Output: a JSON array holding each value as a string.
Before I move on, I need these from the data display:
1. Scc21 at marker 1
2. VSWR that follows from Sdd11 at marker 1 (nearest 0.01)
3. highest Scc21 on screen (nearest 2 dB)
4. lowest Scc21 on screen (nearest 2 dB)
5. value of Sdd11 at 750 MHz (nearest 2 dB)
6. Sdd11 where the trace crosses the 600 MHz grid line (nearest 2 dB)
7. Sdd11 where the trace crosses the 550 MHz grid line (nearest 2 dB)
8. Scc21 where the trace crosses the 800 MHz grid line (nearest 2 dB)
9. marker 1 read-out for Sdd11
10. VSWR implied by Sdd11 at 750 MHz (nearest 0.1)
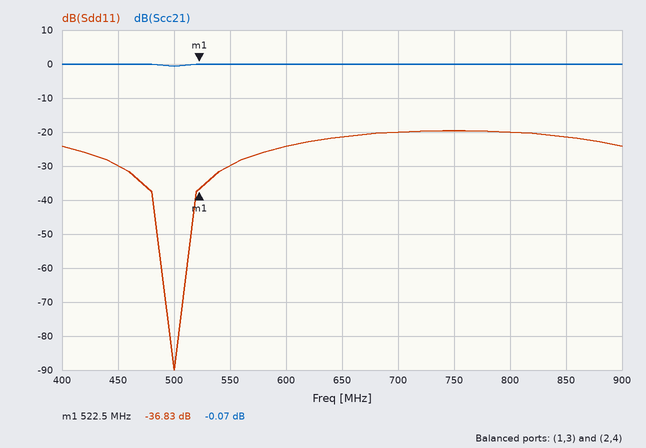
["-0.07 dB", "1.03", "0 dB", "0 dB", "-20 dB", "-24 dB", "-30 dB", "0 dB", "-36.83 dB", "1.2"]
